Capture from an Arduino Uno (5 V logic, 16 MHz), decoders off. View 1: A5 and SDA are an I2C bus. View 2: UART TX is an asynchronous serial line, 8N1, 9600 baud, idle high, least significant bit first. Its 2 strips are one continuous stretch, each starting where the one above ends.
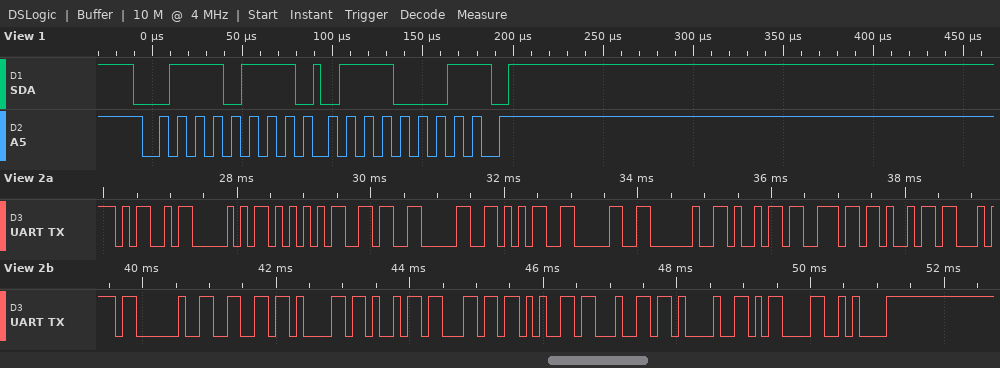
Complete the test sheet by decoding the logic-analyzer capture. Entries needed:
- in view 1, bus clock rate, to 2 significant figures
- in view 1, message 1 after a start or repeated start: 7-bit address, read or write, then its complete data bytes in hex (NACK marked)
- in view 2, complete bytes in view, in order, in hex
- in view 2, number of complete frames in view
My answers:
100 kHz
0x3B read: 71 NACK
4D 50 55 36 30 35 30 20 69 6E 69 74 20 66 61 69 6C 65 64 21 0D 0A
22
